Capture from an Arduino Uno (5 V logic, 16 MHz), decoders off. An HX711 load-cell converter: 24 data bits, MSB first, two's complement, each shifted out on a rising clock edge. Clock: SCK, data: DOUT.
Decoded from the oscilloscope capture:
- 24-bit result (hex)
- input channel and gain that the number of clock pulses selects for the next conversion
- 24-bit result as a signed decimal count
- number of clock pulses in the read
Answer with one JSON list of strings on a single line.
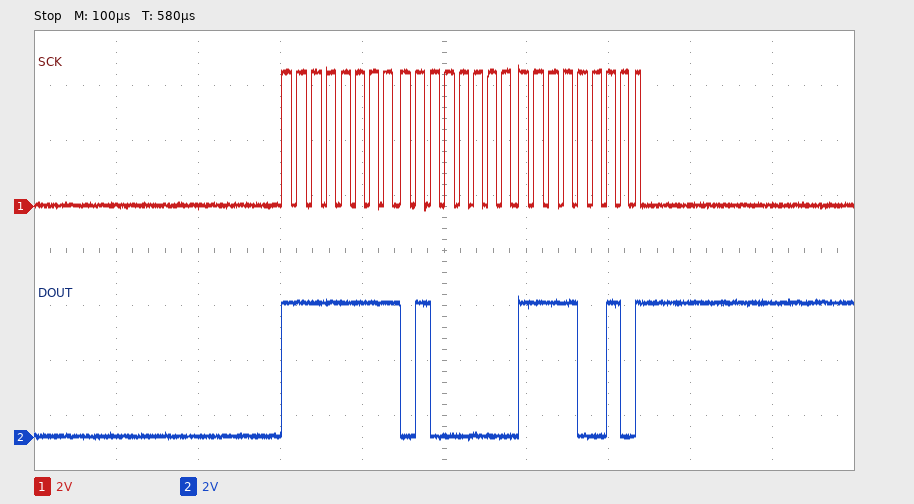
["0xFF40F2", "channel A, gain 128", "-48910", "25"]
